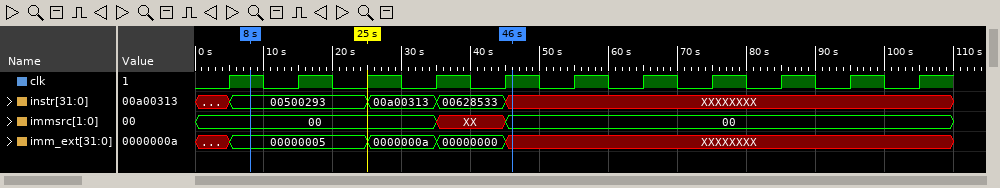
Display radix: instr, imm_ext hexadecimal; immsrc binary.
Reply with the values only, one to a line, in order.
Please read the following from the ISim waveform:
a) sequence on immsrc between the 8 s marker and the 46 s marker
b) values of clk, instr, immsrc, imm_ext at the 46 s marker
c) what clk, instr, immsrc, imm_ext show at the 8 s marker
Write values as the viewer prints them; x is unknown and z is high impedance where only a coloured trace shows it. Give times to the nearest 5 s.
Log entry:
00, XX, 00
clk=1, instr=XXXXXXXX, immsrc=00, imm_ext=XXXXXXXX
clk=1, instr=00500293, immsrc=00, imm_ext=00000005
